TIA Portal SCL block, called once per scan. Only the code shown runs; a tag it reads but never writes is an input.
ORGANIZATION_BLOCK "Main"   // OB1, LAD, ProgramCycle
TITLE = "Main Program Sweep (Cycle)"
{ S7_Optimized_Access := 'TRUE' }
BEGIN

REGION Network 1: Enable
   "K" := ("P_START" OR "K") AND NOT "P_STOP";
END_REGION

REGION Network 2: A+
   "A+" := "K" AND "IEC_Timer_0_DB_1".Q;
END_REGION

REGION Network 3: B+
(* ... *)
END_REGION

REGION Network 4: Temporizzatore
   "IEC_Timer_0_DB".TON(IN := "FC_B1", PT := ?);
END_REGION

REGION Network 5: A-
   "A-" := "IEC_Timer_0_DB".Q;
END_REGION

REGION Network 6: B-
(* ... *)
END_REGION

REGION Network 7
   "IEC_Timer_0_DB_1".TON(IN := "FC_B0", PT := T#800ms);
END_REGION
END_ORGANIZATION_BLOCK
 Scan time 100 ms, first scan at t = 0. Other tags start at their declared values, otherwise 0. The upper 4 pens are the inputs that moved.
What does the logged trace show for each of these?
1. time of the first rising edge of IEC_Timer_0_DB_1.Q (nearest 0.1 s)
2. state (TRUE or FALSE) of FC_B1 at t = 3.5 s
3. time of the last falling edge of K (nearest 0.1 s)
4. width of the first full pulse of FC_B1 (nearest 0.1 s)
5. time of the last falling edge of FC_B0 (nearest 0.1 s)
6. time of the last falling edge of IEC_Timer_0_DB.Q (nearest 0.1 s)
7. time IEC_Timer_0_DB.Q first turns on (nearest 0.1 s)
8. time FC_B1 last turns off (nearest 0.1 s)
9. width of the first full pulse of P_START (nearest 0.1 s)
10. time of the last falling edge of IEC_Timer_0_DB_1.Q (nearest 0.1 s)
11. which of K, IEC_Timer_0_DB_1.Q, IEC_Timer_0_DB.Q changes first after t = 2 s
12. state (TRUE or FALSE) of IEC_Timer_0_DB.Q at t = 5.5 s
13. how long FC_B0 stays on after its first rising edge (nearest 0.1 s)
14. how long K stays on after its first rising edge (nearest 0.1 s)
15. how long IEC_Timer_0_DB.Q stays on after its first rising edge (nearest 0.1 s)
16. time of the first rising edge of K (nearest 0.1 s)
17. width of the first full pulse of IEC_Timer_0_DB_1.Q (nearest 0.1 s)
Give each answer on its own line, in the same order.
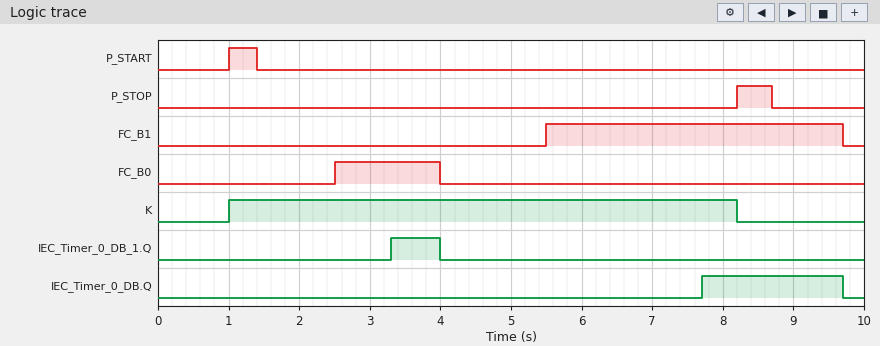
3.3 s
FALSE
8.2 s
4.2 s
4.0 s
9.7 s
7.7 s
9.7 s
0.4 s
4.0 s
IEC_Timer_0_DB_1.Q
FALSE
1.5 s
7.2 s
2.0 s
1.0 s
0.7 s
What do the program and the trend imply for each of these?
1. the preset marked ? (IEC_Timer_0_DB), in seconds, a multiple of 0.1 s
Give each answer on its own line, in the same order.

2.2 s
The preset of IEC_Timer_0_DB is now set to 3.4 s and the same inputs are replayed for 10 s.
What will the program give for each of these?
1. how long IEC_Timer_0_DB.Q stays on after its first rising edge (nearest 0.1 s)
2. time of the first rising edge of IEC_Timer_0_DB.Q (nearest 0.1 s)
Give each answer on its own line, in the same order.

0.8 s
8.9 s
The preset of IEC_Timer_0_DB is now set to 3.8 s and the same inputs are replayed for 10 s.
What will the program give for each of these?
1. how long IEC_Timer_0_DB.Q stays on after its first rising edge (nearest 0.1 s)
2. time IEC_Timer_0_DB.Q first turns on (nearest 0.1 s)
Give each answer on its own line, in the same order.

0.4 s
9.3 s
